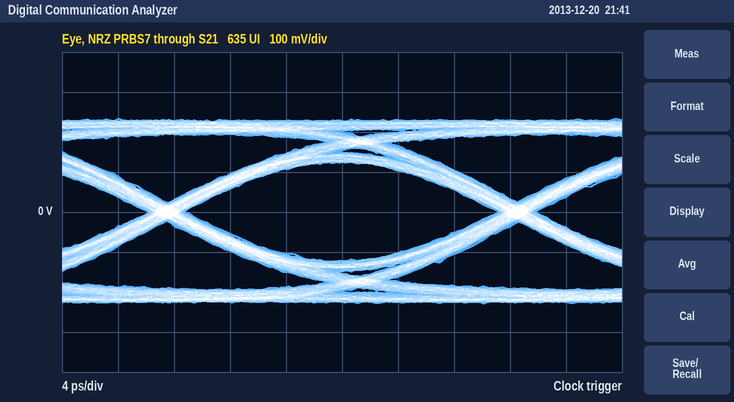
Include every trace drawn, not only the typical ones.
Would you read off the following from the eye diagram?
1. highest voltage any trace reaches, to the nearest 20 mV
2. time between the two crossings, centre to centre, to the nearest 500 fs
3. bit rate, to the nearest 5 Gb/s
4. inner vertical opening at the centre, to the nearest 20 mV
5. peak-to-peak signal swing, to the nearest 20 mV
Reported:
240 mV
25.0 ps
40 Gb/s
240 mV
460 mV
